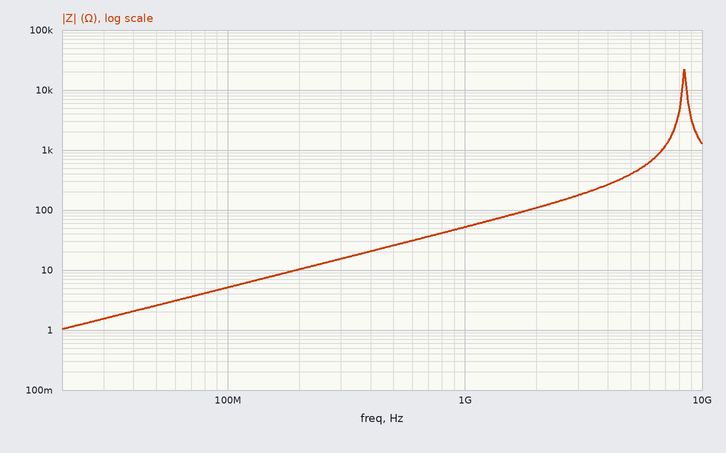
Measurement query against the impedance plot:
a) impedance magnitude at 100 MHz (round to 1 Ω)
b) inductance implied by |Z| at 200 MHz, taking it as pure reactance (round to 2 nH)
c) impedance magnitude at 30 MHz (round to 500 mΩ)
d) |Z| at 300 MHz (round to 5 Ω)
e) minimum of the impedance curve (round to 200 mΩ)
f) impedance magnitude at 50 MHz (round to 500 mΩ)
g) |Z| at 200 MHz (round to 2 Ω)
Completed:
5 Ω
8 nH
1.5 Ω
15 Ω
1.0 Ω
2.5 Ω
10 Ω
